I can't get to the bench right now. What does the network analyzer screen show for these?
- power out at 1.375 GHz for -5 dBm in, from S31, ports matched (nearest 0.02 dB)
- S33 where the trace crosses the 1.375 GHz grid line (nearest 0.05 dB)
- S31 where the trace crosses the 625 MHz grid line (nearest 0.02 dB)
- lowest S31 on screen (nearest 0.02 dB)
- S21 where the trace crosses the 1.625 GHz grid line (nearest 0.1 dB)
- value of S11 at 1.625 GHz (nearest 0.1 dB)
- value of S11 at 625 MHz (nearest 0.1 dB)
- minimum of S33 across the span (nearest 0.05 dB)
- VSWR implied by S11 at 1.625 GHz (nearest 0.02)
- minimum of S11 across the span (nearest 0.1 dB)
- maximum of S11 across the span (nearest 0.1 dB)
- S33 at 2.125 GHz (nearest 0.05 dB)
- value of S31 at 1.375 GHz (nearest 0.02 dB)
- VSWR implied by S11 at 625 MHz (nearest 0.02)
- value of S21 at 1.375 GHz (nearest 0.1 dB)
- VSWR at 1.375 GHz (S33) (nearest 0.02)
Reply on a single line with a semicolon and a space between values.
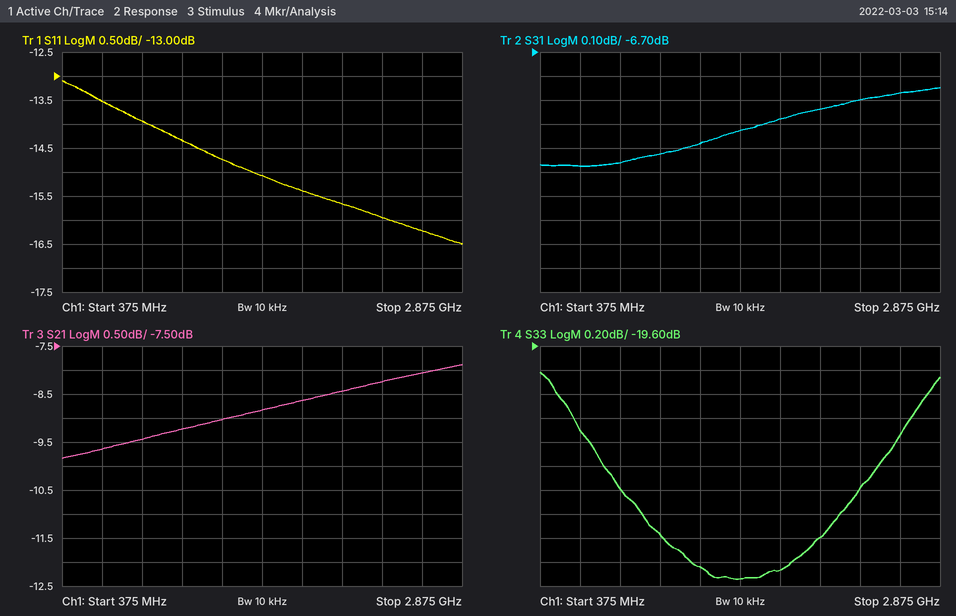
-12.08 dBm; -21.45 dB; -7.18 dB; -7.18 dB; -8.8 dB; -15.1 dB; -13.5 dB; -21.55 dB; 1.42; -16.5 dB; -13.1 dB; -21.20 dB; -7.08 dB; 1.54; -9.0 dB; 1.18
